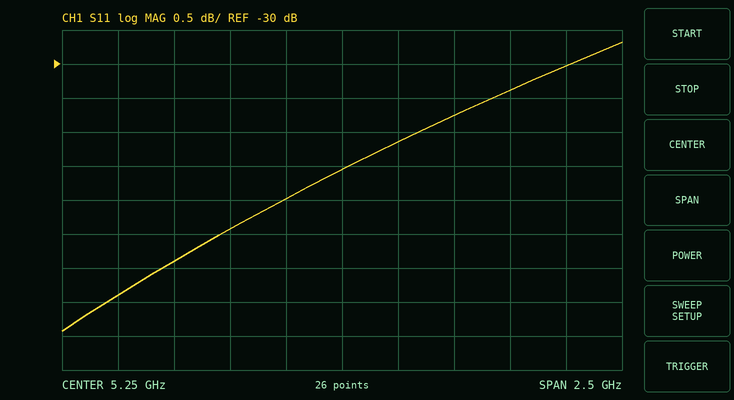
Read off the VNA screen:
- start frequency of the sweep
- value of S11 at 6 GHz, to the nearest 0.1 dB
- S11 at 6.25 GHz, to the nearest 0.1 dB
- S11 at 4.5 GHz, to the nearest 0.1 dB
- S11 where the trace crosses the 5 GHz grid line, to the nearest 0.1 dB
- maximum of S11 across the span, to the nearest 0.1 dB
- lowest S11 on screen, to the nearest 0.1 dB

4 GHz
-30.4 dB
-30.0 dB
-32.9 dB
-32.0 dB
-29.7 dB
-33.9 dB
